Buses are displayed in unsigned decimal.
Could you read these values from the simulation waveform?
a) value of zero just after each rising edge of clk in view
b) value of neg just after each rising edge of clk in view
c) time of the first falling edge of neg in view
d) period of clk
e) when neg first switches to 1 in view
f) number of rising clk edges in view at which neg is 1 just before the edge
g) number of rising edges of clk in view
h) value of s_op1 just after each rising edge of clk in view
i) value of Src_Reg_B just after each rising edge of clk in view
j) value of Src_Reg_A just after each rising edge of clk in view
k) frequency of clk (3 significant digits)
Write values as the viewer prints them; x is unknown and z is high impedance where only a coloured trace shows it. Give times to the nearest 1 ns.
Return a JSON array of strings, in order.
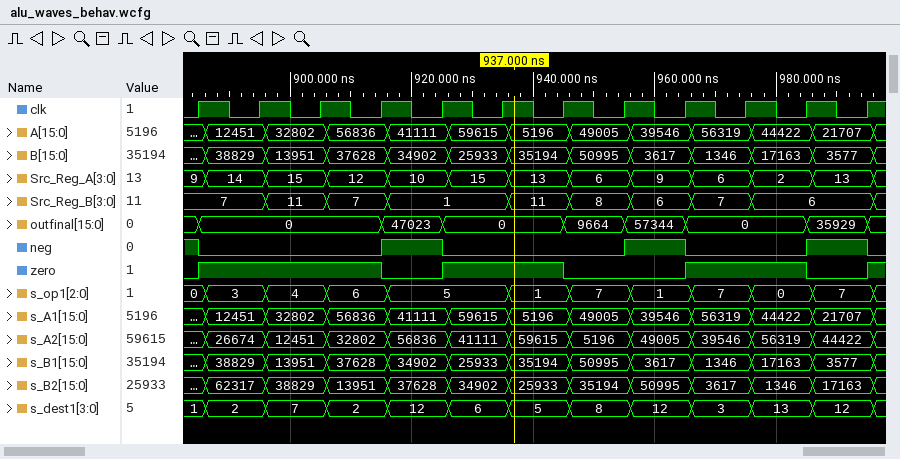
["1 1 1 0 1 1 0 0 1 1 0 1", "0 0 0 1 0 0 0 1 0 0 1 0", "885 ns", "10 ns", "915 ns", "4", "12", "0, 3, 4, 6, 5, 5, 1, 7, 1, 7, 0, 7", "7, 7, 11, 7, 1, 1, 11, 8, 6, 7, 6, 6", "9, 14, 15, 12, 10, 15, 13, 6, 9, 6, 2, 13", "100 MHz"]
